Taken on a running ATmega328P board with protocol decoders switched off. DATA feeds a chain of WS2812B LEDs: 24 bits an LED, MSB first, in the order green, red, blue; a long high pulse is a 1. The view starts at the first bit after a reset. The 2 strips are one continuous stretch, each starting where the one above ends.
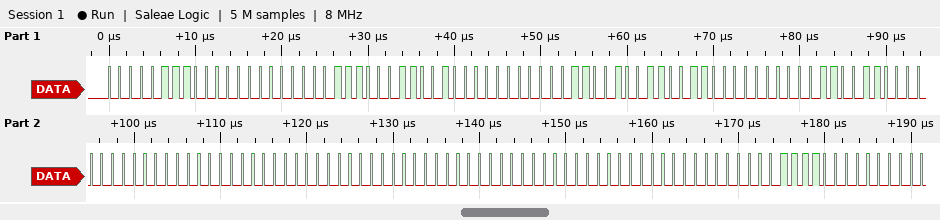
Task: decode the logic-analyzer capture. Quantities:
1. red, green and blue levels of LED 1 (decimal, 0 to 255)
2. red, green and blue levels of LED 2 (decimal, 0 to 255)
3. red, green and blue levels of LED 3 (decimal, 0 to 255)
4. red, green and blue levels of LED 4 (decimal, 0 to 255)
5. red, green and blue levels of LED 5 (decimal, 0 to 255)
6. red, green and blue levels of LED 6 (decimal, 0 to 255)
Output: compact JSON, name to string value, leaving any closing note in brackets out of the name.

{"red, green and blue levels of LED 1": "0, 7, 7", "red, green and blue levels of LED 2": "0, 25, 25", "red, green and blue levels of LED 3": "0, 51, 51", "red, green and blue levels of LED 4": "0, 0, 0", "red, green and blue levels of LED 5": "0, 0, 0", "red, green and blue levels of LED 6": "0, 0, 15"}
